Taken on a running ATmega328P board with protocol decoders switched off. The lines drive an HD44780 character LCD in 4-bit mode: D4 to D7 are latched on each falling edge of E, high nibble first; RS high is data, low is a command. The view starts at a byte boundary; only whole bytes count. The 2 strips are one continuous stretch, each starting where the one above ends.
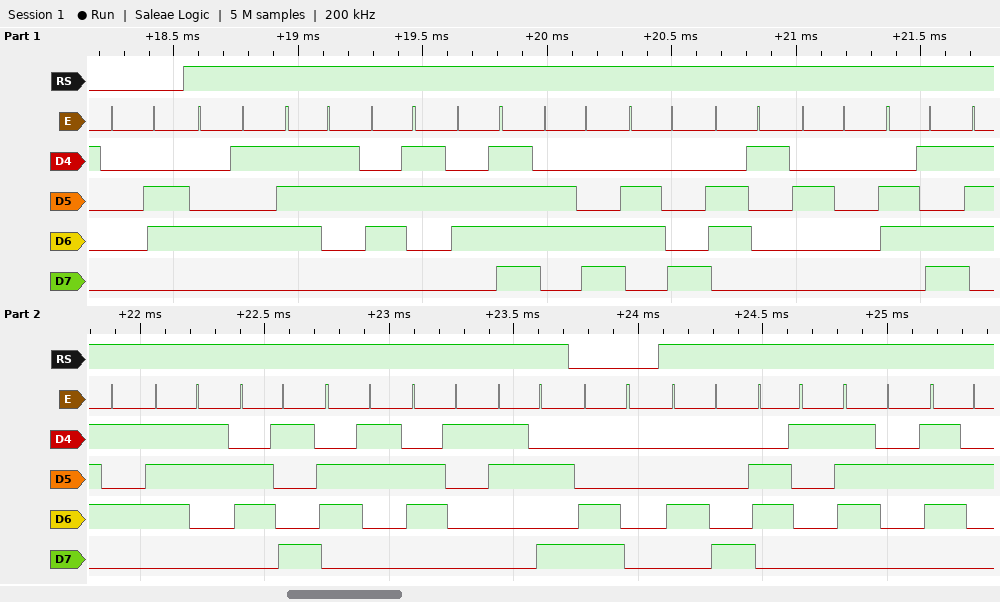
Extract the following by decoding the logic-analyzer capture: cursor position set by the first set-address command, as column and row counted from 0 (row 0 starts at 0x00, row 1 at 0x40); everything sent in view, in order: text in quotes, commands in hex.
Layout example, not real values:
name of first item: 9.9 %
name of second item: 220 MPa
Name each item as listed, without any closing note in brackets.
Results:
cursor position set by the first set-address command, as column and row counted from 0: column 0, row 1
everything sent in view, in order: text in quotes, commands in hex: 0x06 "Escolha musica:" 0xC0 "Harr"
